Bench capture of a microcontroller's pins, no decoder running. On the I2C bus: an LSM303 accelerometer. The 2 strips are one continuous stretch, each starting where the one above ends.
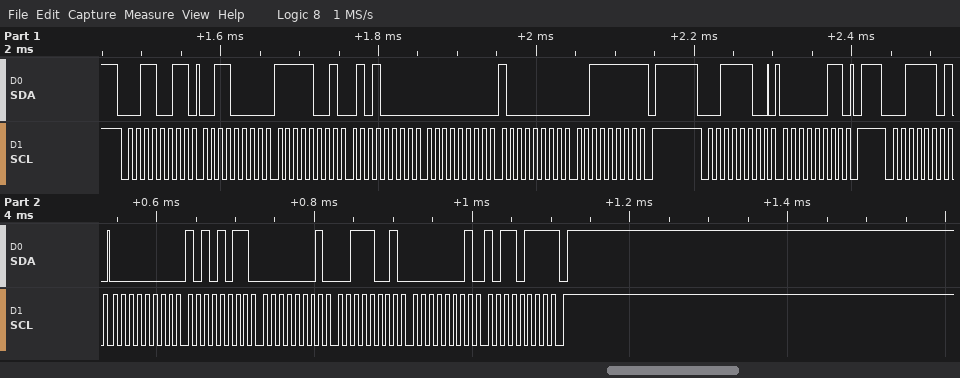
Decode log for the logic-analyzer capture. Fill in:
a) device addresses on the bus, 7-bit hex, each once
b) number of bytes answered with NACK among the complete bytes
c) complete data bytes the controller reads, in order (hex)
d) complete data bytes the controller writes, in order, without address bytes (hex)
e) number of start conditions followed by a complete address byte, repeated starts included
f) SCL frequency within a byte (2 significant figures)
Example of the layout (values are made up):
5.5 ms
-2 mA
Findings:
0x19 0x1E
2
30 F9 50 00 80 3F 00 AB 01 39 01 B7
03
3
100 kHz
